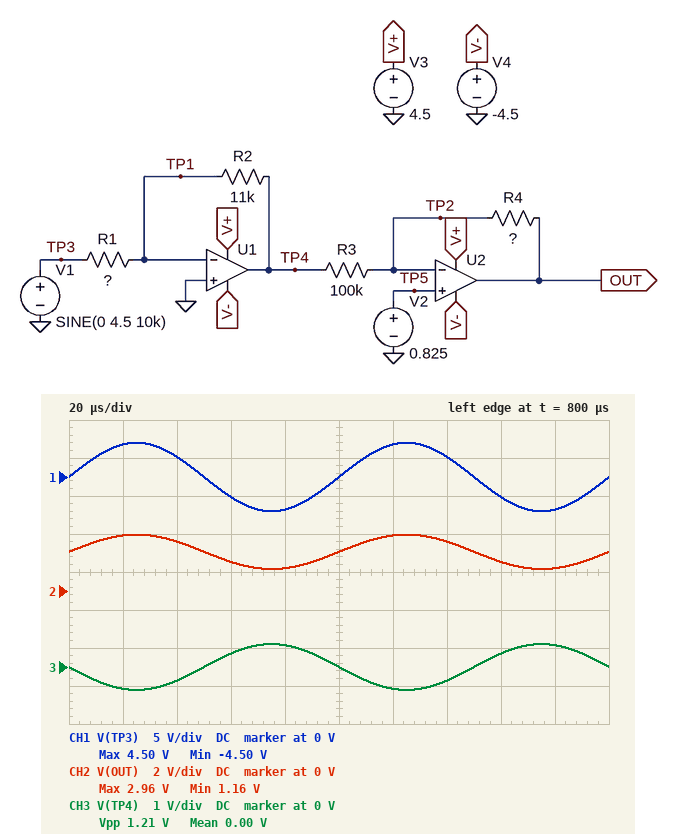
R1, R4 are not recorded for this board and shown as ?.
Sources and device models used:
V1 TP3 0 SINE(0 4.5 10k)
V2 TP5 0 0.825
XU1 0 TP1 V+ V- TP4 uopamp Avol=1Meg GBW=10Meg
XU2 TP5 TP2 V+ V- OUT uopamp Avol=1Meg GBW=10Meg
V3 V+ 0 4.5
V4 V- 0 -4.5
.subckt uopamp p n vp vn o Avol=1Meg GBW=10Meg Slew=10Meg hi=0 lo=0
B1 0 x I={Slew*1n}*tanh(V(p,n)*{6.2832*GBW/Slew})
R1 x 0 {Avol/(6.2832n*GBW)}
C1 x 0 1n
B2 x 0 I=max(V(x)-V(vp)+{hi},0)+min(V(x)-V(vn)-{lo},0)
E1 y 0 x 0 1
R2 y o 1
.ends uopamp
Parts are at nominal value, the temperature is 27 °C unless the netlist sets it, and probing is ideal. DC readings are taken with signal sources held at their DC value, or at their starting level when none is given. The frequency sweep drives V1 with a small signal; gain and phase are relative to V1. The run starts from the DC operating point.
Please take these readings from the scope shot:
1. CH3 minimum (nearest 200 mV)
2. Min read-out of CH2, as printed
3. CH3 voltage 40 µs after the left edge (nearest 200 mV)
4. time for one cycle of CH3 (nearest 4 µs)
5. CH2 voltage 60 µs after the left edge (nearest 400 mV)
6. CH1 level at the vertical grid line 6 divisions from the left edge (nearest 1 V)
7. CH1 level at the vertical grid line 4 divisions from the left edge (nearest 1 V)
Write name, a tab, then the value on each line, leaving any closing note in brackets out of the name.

CH3 minimum	-600 mV
Min read-out of CH2, as printed	1.16 V
CH3 voltage 40 µs after the left edge	-400 mV
time for one cycle of CH3	100 µs
CH2 voltage 60 µs after the left edge	1.6 V
CH1 level at the vertical grid line 6 divisions from the left edge	4 V
CH1 level at the vertical grid line 4 divisions from the left edge	-4 V
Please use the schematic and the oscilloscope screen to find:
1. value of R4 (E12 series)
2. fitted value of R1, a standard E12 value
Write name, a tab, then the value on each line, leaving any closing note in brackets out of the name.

value of R4	150 kΩ
fitted value of R1, a standard E12 value	82 kΩ
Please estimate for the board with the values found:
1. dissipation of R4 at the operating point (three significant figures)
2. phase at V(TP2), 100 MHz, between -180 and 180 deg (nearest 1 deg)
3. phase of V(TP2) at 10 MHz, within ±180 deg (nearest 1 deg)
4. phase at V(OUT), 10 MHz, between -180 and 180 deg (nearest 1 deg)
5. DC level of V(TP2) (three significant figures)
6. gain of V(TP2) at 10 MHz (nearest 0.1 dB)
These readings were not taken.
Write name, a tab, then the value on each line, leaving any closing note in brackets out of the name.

dissipation of R4 at the operating point	10.2 µW
phase at V(TP2), 100 MHz, between -180 and 180 deg	97 deg
phase of V(TP2) at 10 MHz, within ±180 deg	153 deg
phase at V(OUT), 10 MHz, between -180 and 180 deg	-117 deg
DC level of V(TP2)	825 mV
gain of V(TP2) at 10 MHz	-26.1 dB
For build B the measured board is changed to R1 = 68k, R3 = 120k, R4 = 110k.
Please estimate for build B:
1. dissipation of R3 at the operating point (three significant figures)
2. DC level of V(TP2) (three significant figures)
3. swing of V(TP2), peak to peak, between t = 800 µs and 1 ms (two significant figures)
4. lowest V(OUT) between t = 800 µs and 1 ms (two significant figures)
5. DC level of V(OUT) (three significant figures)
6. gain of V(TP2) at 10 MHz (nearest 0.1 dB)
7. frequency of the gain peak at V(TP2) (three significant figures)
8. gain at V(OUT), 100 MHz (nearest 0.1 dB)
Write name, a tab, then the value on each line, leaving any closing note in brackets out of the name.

dissipation of R3 at the operating point	5.67 µW
DC level of V(TP2)	825 mV
swing of V(TP2), peak to peak, between t = 800 µs and 1 ms	1.3 mV
lowest V(OUT) between t = 800 µs and 1 ms	910 mV
DC level of V(OUT)	1.58 V
gain of V(TP2) at 10 MHz	-27.0 dB
frequency of the gain peak at V(TP2)	6.70 MHz
gain at V(OUT), 100 MHz	-63.6 dB
